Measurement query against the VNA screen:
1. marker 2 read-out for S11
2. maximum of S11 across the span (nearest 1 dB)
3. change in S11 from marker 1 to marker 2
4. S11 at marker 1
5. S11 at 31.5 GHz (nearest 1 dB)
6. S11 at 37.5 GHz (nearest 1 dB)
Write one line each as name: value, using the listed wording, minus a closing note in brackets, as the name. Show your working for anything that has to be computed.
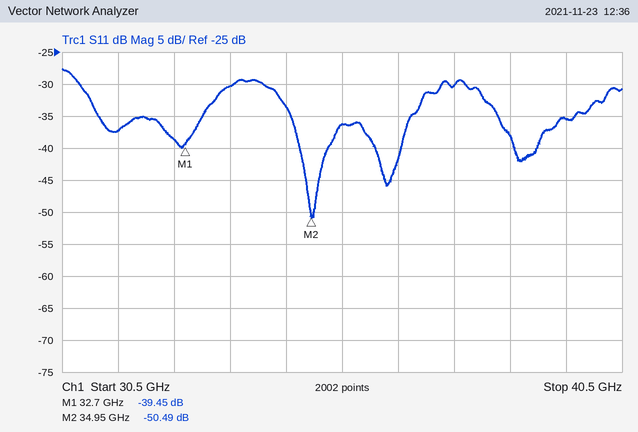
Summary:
marker 2 read-out for S11: -50.49 dB
maximum of S11 across the span: -28 dB
change in S11 from marker 1 to marker 2: -50.49 − (-39.45) = -11.04 dB
S11 at marker 1: -39.45 dB
S11 at 31.5 GHz: -37 dB
S11 at 37.5 GHz: -30 dB
